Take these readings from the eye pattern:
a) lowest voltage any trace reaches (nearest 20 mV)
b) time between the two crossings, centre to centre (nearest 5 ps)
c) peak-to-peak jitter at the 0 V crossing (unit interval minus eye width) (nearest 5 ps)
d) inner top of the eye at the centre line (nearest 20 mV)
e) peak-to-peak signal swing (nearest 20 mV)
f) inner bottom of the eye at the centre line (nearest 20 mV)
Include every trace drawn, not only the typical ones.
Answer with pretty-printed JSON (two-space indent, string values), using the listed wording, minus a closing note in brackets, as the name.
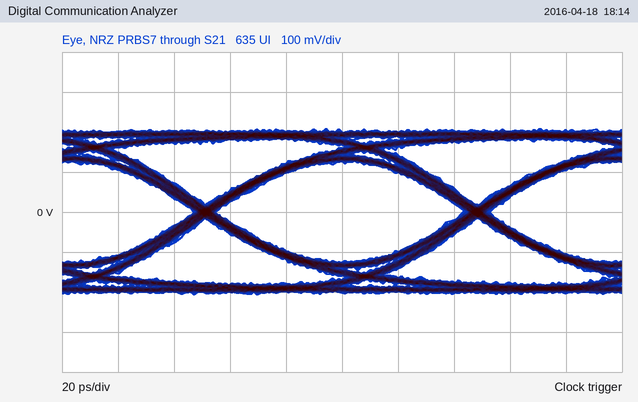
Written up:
{
  "lowest voltage any trace reaches": "-200 mV",
  "time between the two crossings, centre to centre": "95 ps",
  "peak-to-peak jitter at the 0 V crossing (unit interval minus eye width)": "10 ps",
  "inner top of the eye at the centre line": "120 mV",
  "peak-to-peak signal swing": "420 mV",
  "inner bottom of the eye at the centre line": "-120 mV"
}
